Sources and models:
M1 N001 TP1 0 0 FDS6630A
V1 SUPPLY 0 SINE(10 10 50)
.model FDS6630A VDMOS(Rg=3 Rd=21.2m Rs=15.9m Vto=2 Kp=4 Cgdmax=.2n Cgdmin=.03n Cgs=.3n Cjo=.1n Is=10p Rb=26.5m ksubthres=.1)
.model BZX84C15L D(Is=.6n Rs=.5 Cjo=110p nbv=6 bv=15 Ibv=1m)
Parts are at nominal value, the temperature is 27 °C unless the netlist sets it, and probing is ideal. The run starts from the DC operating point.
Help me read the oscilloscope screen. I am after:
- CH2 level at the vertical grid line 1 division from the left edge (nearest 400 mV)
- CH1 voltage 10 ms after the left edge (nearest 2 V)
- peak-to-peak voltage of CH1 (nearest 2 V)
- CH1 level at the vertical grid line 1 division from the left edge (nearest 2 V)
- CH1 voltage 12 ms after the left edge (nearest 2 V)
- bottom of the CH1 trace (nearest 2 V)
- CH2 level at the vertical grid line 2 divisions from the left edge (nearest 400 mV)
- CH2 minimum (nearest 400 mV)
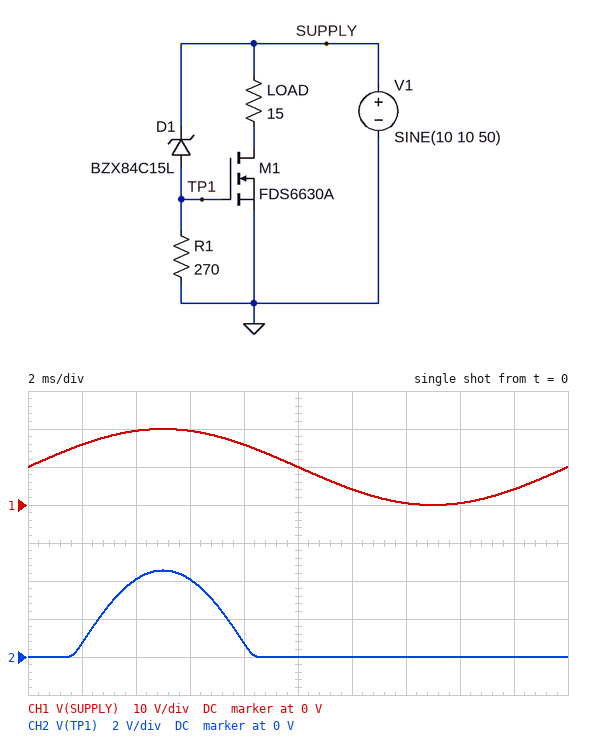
800 mV
10 V
20 V
16 V
4 V
0 V
4.0 V
0 V
